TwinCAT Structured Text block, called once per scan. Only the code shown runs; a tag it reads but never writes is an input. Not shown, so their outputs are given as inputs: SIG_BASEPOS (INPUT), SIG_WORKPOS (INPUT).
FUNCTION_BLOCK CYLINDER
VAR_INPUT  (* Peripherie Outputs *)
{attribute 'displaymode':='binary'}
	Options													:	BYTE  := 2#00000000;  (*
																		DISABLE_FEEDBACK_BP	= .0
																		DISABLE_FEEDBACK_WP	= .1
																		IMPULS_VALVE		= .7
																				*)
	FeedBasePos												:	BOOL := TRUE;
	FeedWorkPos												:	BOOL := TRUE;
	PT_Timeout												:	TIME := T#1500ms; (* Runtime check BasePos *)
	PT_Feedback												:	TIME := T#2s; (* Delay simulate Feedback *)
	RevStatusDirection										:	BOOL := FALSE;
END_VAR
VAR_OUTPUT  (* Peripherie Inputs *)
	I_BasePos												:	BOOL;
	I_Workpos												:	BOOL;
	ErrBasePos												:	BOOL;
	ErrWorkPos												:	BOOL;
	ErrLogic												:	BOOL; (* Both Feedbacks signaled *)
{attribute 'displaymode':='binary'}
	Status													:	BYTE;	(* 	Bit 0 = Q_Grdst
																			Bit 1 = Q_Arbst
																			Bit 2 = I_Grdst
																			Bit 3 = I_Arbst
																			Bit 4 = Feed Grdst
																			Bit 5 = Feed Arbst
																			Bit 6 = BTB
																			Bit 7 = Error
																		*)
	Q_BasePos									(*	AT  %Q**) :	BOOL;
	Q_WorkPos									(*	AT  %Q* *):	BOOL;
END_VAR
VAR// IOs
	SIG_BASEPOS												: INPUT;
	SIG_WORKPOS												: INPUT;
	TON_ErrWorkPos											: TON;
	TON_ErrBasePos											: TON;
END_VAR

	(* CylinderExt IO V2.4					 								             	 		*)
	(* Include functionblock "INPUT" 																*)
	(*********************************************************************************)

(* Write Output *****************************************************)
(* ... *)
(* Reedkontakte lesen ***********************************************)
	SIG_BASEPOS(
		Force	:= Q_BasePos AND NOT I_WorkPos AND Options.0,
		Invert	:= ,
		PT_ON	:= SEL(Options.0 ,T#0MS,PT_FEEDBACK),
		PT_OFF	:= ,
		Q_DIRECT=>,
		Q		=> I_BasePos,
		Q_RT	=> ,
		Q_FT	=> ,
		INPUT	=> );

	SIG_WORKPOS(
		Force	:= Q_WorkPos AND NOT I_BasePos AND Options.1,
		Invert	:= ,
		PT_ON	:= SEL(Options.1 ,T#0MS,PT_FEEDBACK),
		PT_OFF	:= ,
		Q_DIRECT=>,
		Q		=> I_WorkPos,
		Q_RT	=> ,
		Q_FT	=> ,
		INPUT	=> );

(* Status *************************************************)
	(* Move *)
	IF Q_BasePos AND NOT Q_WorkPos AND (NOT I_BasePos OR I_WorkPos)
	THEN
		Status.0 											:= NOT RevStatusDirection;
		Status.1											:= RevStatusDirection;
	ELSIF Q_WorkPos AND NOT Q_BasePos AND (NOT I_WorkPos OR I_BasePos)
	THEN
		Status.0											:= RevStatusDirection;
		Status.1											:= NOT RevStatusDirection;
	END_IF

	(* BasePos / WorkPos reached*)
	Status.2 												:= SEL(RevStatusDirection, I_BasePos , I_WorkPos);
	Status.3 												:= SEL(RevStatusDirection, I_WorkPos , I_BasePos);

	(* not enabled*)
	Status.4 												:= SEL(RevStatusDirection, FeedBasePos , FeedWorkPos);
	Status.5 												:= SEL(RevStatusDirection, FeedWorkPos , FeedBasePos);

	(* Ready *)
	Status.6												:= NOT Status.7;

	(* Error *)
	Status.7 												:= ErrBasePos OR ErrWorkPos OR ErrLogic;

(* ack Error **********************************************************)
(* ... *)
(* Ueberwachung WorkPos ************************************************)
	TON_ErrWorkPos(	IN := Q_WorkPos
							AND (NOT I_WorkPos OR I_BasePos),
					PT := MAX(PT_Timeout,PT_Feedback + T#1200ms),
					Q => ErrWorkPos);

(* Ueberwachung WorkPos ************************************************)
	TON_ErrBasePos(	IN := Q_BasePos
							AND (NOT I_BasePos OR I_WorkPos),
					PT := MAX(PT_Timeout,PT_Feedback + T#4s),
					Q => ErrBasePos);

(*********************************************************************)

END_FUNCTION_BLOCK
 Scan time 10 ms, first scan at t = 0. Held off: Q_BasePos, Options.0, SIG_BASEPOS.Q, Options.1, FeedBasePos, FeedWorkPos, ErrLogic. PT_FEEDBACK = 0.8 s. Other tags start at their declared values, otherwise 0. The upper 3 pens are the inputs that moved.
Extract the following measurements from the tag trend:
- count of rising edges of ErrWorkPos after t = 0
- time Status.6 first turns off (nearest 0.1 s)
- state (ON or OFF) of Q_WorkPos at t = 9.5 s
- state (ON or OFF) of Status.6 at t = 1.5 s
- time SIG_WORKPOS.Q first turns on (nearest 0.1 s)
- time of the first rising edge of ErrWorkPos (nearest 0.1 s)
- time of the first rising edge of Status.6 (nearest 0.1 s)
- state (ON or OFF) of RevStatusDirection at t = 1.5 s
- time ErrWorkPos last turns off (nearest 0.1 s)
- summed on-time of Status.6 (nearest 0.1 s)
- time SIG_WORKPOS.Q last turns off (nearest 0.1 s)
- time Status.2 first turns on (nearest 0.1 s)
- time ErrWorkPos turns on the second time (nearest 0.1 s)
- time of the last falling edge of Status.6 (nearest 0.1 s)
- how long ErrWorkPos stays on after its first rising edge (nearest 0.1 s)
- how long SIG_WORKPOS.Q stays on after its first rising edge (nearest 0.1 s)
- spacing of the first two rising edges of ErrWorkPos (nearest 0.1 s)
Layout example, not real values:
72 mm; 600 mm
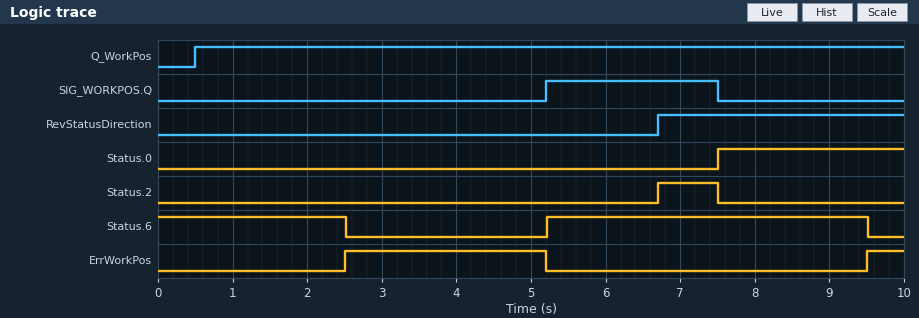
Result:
2; 2.5 s; ON; ON; 5.2 s; 2.5 s; 5.2 s; OFF; 5.2 s; 6.8 s; 7.5 s; 6.7 s; 9.5 s; 9.5 s; 2.7 s; 2.3 s; 7.0 s
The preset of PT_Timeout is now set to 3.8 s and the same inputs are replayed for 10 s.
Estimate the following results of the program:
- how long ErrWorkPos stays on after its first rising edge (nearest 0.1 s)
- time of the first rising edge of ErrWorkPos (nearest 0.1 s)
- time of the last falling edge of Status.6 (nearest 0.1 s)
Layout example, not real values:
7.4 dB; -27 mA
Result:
0.9 s; 4.3 s; 4.3 s
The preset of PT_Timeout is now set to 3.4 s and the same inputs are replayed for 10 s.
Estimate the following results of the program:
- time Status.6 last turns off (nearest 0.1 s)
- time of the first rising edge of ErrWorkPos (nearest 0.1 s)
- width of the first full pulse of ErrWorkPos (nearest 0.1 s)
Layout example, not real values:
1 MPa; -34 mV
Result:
3.9 s; 3.9 s; 1.3 s
